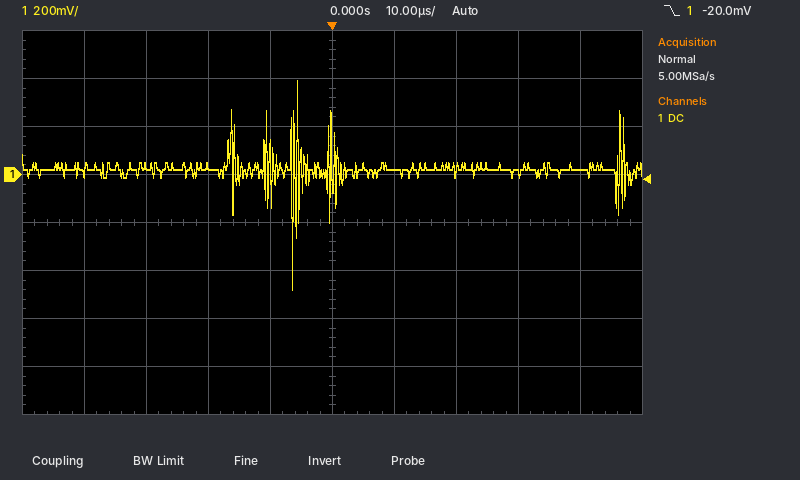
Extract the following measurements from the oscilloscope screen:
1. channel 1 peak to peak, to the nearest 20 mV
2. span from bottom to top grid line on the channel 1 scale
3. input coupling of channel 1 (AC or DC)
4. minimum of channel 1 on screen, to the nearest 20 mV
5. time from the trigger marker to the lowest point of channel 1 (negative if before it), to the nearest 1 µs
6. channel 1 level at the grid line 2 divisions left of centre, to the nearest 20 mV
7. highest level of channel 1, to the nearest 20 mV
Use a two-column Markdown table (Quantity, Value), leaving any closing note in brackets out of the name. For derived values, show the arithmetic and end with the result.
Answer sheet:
| Quantity | Value |
|---|---|
| channel 1 peak to peak, to the nearest 20 mV | 400 mV − (-480 mV) = 880 mV |
| span from bottom to top grid line on the channel 1 scale | 1.6 V |
| input coupling of channel 1 | DC |
| minimum of channel 1 on screen, to the nearest 20 mV | -480 mV |
| time from the trigger marker to the lowest point of channel 1 (negative if before it), to the nearest 1 µs | -6 µs |
| channel 1 level at the grid line 2 divisions left of centre, to the nearest 20 mV | 40 mV |
| highest level of channel 1, to the nearest 20 mV | 400 mV |
